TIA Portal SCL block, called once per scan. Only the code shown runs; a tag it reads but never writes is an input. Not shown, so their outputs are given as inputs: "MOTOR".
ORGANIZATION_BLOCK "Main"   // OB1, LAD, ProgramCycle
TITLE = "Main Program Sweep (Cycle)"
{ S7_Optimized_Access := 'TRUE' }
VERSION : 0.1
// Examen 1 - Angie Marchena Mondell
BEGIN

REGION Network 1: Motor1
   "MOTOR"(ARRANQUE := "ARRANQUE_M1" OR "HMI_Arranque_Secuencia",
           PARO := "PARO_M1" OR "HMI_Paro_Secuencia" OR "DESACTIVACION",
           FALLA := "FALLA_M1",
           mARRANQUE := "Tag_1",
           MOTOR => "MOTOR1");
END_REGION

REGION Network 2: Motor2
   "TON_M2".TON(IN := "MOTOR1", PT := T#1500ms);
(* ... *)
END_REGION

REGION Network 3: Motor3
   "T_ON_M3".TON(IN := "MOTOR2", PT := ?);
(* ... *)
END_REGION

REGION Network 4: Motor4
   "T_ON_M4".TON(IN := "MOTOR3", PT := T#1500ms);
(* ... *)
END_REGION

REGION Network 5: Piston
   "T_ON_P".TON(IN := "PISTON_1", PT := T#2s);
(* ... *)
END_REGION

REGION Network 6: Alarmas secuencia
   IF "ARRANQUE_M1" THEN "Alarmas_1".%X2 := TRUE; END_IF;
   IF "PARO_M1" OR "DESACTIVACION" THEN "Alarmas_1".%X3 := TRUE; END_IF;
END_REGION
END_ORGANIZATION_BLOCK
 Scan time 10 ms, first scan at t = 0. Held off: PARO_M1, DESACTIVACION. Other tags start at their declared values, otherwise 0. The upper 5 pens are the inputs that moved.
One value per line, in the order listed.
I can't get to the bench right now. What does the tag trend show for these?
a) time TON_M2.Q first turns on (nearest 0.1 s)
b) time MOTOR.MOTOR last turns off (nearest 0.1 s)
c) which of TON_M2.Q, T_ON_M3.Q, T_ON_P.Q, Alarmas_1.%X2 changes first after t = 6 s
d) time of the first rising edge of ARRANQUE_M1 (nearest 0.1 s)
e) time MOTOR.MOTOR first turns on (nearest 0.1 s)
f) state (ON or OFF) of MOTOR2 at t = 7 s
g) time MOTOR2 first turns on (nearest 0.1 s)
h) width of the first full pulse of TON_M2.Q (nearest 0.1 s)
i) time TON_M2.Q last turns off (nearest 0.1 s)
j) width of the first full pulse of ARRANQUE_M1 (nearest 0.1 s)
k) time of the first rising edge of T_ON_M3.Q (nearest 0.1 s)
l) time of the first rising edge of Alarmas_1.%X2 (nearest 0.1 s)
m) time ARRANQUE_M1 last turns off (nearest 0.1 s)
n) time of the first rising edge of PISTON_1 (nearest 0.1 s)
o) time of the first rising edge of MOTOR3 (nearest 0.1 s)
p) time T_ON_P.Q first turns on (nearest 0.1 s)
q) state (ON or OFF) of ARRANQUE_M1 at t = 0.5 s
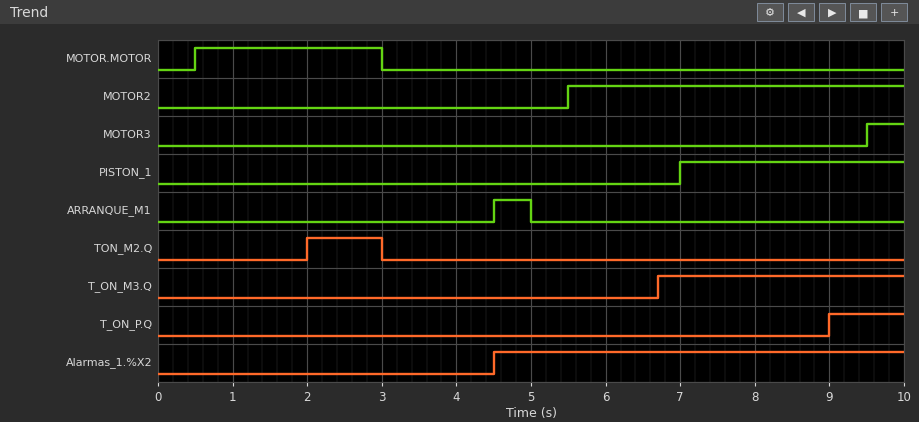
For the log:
2.0 s
3.0 s
T_ON_M3.Q
4.5 s
0.5 s
ON
5.5 s
1.0 s
3.0 s
0.5 s
6.7 s
4.5 s
5.0 s
7.0 s
9.5 s
9.0 s
OFF
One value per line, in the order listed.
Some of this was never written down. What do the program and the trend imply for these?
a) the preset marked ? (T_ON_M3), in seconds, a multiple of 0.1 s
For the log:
1.2 s
